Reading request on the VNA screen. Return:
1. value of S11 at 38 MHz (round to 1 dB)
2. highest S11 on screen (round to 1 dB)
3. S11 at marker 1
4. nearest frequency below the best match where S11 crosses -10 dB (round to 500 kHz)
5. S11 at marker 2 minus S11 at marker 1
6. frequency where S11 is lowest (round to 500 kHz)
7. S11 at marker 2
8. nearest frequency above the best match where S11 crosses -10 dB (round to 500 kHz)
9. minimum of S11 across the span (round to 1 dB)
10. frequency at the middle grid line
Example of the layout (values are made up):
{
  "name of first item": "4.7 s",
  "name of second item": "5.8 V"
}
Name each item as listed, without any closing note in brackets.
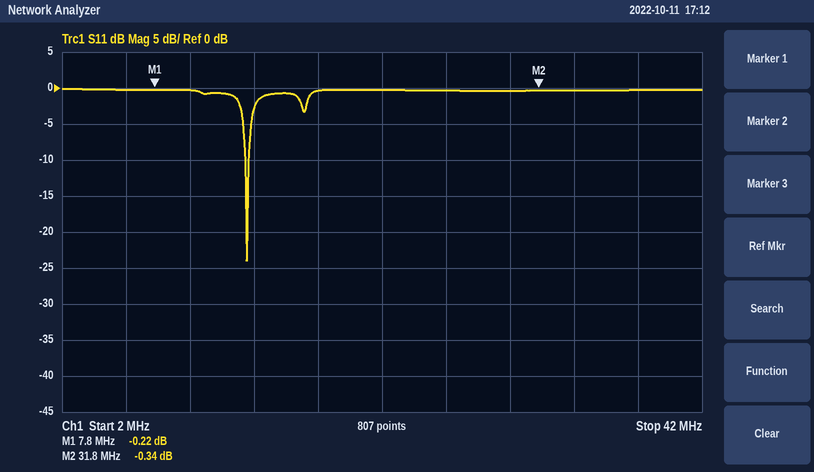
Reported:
{
  "value of S11 at 38 MHz": "0 dB",
  "highest S11 on screen": "0 dB",
  "S11 at marker 1": "-0.22 dB",
  "nearest frequency below the best match where S11 crosses -10 dB": "13.5 MHz",
  "S11 at marker 2 minus S11 at marker 1": "-0.12 dB",
  "frequency where S11 is lowest": "13.5 MHz",
  "S11 at marker 2": "-0.34 dB",
  "nearest frequency above the best match where S11 crosses -10 dB": "13.5 MHz",
  "minimum of S11 across the span": "-24 dB",
  "frequency at the middle grid line": "22 MHz"
}
